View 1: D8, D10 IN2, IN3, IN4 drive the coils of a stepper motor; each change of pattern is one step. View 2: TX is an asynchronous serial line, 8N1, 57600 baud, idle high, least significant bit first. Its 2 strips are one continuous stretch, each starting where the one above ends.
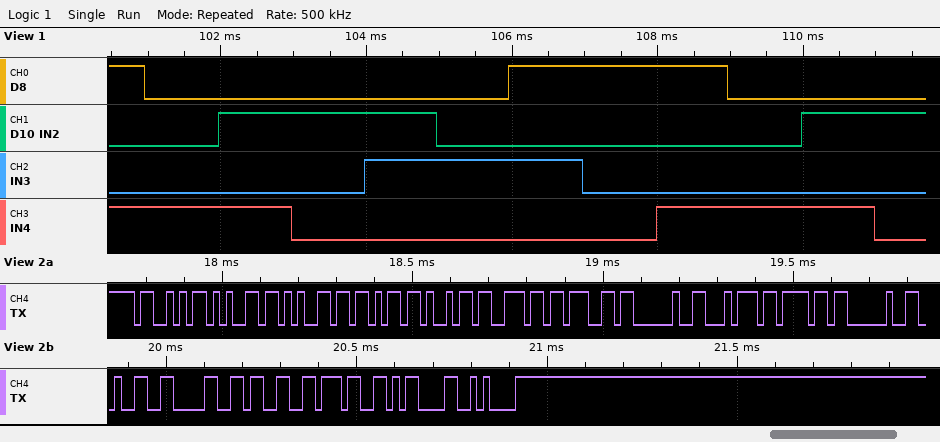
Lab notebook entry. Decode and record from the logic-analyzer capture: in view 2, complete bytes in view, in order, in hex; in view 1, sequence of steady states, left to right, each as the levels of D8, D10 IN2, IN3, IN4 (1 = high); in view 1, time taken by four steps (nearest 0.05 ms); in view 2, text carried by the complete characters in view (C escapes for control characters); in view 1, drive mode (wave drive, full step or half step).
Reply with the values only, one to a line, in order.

53 65 65 6B 69 6E 67 20 74 6F 20 32 30 33 37 0D 0A
1001 0001 0101 0100 0110 0010 1010 1000 1001 0001 0101 0100
4.00 ms
"Seeking to 2037\r\n"
half step
